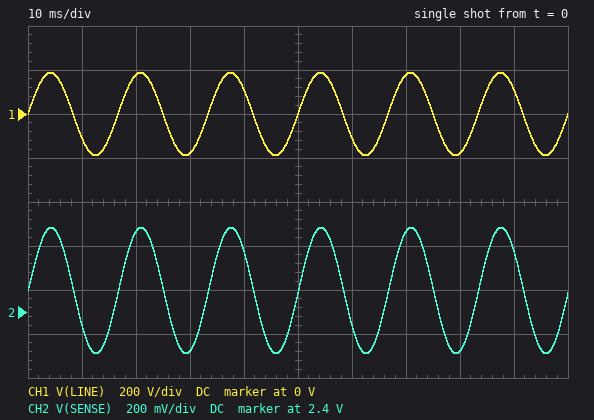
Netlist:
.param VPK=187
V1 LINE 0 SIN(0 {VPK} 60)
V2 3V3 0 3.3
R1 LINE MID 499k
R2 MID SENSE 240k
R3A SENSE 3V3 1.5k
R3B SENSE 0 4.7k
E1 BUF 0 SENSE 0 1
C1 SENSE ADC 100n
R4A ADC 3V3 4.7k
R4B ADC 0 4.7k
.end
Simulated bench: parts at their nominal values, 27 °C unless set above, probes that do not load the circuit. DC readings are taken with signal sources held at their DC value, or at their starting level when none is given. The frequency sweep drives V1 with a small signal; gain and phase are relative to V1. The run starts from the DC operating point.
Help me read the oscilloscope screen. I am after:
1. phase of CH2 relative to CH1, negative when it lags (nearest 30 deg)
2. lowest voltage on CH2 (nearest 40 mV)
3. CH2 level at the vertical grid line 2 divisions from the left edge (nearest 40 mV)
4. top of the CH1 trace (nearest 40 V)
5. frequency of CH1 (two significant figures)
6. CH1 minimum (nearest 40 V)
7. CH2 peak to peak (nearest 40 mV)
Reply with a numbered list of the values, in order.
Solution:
1. 0 deg
2. 2.20 V
3. 2.76 V
4. 200 V
5. 60 Hz
6. -200 V
7. 560 mV
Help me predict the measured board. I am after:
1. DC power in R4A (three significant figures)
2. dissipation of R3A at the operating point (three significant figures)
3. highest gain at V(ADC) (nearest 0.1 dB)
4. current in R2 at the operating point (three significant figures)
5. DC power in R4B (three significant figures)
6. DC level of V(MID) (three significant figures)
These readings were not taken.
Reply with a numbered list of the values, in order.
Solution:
1. 579 µW
2. 429 µW
3. -59.7 dB
4. 3.38 µA
5. 579 µW
6. 1.69 V
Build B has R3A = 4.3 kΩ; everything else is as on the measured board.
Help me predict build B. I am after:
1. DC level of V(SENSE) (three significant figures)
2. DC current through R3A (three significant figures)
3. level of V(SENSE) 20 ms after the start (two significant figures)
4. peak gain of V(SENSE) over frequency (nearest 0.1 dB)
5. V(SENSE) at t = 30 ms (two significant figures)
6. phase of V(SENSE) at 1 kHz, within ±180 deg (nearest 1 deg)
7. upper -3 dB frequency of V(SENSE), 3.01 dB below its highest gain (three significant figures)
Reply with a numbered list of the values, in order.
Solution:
1. 1.72 V
2. 368 µA
3. 2.2 V
4. -50.4 dB
5. 1.2 V
6. -15 deg
7. 503 Hz
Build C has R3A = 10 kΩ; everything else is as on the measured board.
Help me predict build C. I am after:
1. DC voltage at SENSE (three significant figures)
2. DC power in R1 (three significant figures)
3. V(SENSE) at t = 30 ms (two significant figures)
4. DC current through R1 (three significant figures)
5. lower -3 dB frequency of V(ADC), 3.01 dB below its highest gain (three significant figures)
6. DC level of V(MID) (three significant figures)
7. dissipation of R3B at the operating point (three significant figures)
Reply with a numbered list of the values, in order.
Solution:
1. 1.05 V
2. 1.01 µW
3. 270 mV
4. 1.42 µA
5. 288 Hz
6. 709 mV
7. 235 µW
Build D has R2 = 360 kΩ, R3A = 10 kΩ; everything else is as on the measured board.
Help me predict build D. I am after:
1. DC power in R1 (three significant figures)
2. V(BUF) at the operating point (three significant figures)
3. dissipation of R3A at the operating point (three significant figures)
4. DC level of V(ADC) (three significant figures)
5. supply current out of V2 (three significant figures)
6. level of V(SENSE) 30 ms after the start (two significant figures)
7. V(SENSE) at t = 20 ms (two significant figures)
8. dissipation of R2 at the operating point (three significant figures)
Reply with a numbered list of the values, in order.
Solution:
1. 747 nW
2. 1.05 V
3. 506 µW
4. 1.65 V
5. 576 µA
6. 380 mV
7. 1.7 V
8. 539 nW
